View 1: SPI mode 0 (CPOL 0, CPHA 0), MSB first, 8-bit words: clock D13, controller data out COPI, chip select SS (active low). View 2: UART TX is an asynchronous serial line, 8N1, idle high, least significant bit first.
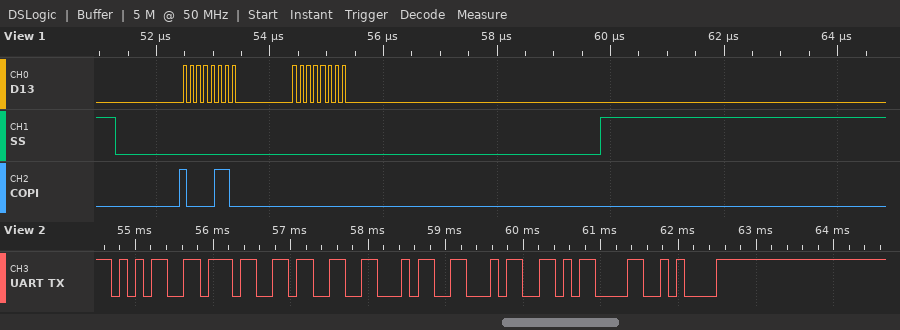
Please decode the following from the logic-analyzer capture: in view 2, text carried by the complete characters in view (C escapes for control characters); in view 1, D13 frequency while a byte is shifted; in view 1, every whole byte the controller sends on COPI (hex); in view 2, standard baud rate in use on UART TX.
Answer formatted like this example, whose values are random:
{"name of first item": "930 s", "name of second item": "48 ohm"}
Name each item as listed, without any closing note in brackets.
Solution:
{"in view 2, text carried by the complete characters in view": "\"57344\\r\\n\"", "in view 1, D13 frequency while a byte is shifted": "8 MHz", "in view 1, every whole byte the controller sends on COPI": "86 00", "in view 2, standard baud rate in use on UART TX": "9600 baud"}
